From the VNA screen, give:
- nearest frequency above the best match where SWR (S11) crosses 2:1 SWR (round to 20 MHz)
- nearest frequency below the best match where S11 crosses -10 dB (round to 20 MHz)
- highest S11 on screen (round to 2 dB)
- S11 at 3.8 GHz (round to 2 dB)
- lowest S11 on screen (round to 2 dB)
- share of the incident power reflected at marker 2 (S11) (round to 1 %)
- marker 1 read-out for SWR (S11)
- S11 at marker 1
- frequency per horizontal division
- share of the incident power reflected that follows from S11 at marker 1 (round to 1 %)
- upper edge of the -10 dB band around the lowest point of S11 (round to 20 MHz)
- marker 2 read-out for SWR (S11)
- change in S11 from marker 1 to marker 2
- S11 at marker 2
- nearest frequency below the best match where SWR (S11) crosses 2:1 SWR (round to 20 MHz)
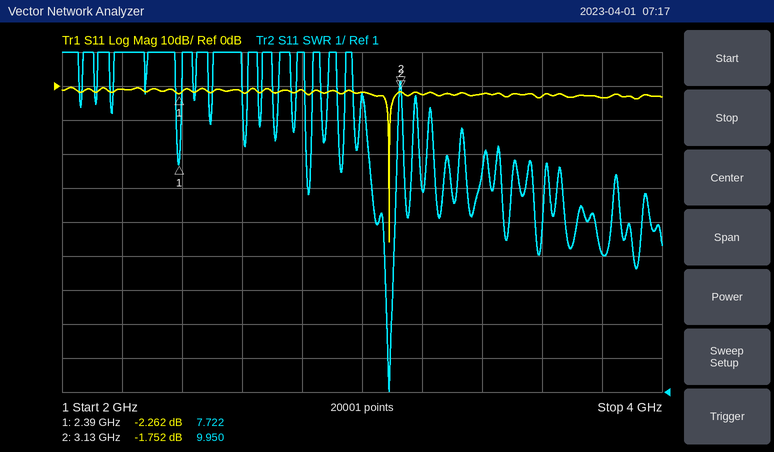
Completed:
3.10 GHz
3.08 GHz
0 dB
-4 dB
-46 dB
67 %
7.722
-2.262 dB
200 MHz
59 %
3.10 GHz
9.950
0.510 dB
-1.752 dB
3.08 GHz
